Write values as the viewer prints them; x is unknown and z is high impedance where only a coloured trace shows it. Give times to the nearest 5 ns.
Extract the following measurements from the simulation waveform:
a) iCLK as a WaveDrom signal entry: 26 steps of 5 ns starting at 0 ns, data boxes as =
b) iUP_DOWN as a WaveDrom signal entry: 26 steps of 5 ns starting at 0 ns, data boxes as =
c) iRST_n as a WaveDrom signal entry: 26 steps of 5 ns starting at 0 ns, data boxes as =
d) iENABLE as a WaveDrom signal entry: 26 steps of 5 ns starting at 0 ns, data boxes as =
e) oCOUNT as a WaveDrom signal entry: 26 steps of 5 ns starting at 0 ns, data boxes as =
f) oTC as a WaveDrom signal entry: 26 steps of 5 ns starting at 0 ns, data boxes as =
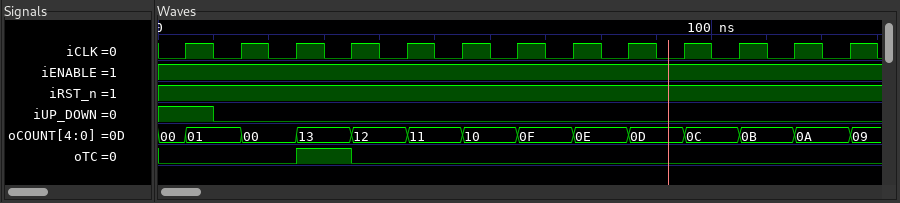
{name: 'iCLK', wave: '01010101010101010101010101'}
{name: 'iUP_DOWN', wave: '1.0.......................'}
{name: 'iRST_n', wave: '1.........................'}
{name: 'iENABLE', wave: '1.........................'}
{name: 'oCOUNT', wave: '==.=.=.=.=.=.=.=.=.=.=.=.=', data: '00 01 00 13 12 11 10 0F 0E 0D 0C 0B 0A 09'}
{name: 'oTC', wave: '0....1.0..................'}
